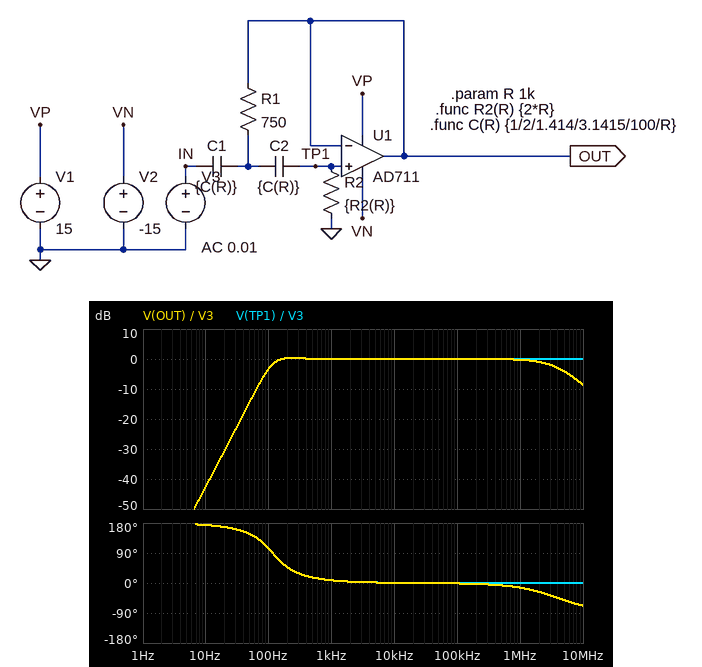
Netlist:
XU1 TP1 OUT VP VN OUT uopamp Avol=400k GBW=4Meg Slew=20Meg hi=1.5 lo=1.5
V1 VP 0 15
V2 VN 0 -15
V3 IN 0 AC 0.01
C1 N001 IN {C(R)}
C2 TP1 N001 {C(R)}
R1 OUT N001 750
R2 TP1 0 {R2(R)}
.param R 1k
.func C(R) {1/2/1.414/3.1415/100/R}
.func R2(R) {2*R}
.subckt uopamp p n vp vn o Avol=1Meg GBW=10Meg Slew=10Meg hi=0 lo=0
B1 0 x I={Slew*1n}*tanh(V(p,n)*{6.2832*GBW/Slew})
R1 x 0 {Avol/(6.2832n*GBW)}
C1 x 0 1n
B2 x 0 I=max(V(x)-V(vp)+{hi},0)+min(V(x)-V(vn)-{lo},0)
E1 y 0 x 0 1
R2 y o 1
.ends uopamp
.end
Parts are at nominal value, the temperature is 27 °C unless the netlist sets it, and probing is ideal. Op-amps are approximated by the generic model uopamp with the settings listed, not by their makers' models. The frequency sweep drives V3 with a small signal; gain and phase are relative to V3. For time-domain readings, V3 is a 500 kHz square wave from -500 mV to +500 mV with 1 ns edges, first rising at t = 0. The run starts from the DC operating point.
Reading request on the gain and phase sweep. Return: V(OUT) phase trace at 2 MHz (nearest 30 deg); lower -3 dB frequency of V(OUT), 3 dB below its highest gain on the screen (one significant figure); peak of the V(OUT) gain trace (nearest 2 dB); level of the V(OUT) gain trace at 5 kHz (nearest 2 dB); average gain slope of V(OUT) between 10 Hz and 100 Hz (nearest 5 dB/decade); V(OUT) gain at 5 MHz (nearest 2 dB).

-30 deg
100 Hz
0 dB
0 dB
40 dB/decade
-4 dB
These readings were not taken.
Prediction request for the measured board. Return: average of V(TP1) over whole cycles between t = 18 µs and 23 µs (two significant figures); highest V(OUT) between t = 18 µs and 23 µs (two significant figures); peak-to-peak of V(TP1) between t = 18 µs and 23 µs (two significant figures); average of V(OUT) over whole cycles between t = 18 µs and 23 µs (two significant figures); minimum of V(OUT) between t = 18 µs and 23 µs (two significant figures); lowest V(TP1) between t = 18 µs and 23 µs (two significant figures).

490 mV
990 mV
1.0 V
490 mV
-9.7 mV
-9.8 mV
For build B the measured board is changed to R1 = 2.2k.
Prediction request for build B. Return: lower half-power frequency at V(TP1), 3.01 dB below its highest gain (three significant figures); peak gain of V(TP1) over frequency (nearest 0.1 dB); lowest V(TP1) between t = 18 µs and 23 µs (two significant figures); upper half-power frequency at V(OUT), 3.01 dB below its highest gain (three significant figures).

112 Hz
0 dB
-9.7 mV
4.00 MHz
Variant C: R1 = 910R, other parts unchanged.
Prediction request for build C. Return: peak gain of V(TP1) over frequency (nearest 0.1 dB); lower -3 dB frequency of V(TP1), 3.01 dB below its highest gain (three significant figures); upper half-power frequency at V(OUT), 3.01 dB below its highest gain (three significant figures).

0 dB
101 Hz
3.96 MHz
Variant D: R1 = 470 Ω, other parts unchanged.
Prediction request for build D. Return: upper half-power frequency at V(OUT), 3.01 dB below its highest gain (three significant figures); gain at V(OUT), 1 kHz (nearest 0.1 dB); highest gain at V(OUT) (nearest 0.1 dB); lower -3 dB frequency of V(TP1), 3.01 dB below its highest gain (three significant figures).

2.64 MHz
0.1 dB
1.4 dB
124 Hz
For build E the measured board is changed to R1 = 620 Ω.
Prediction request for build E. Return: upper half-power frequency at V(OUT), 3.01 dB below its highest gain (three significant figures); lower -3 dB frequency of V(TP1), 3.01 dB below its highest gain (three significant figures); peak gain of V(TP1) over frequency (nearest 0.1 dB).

3.37 MHz
111 Hz
0.7 dB
